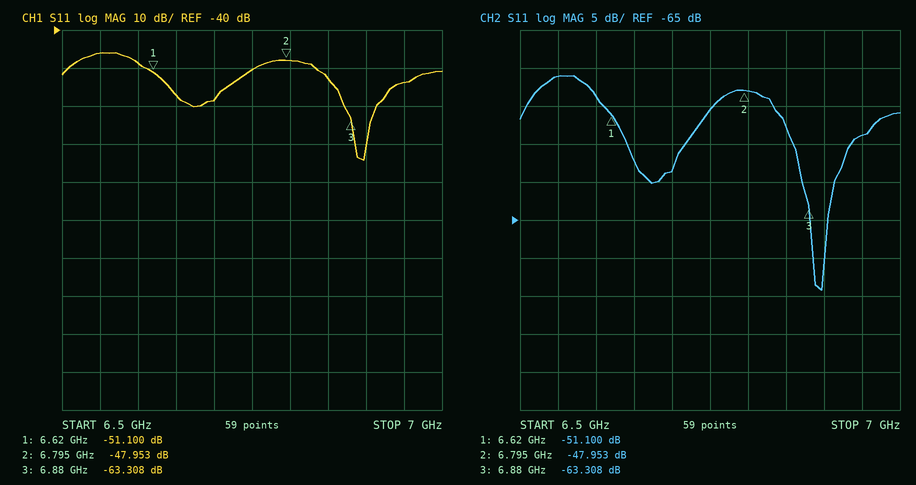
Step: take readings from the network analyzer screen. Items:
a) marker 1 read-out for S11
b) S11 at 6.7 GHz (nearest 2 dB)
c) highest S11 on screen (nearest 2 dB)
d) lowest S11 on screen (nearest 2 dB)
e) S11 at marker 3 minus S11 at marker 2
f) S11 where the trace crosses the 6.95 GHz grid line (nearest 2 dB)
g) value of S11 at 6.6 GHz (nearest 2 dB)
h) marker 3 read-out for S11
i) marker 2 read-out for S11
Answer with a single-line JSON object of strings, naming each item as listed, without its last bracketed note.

{"marker 1 read-out for S11": "-51.100 dB", "S11 at 6.7 GHz": "-58 dB", "highest S11 on screen": "-46 dB", "lowest S11 on screen": "-74 dB", "S11 at marker 3 minus S11 at marker 2": "-15.355 dB", "S11 where the trace crosses the 6.95 GHz grid line": "-54 dB", "value of S11 at 6.6 GHz": "-48 dB", "marker 3 read-out for S11": "-63.308 dB", "marker 2 read-out for S11": "-47.953 dB"}
